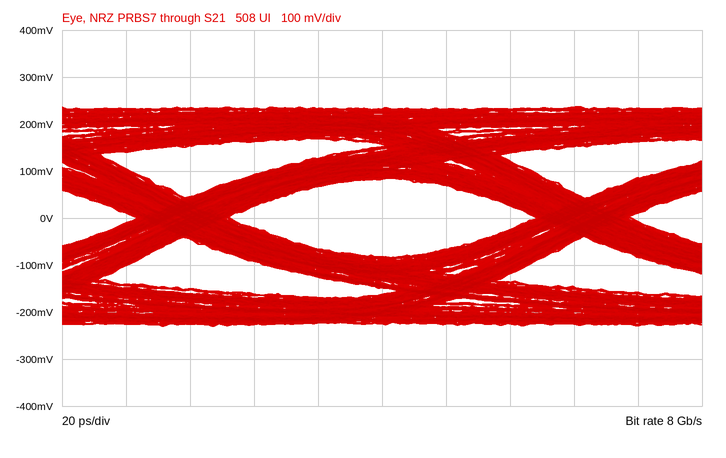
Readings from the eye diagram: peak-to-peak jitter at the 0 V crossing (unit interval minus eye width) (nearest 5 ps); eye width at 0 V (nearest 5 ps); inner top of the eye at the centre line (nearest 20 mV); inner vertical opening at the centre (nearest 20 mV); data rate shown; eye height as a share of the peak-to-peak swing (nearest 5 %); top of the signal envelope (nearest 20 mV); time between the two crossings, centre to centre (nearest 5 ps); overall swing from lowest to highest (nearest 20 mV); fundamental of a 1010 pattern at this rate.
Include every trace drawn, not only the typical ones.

30 ps
95 ps
80 mV
160 mV
8 Gb/s
35 %
240 mV
125 ps
460 mV
4 GHz
